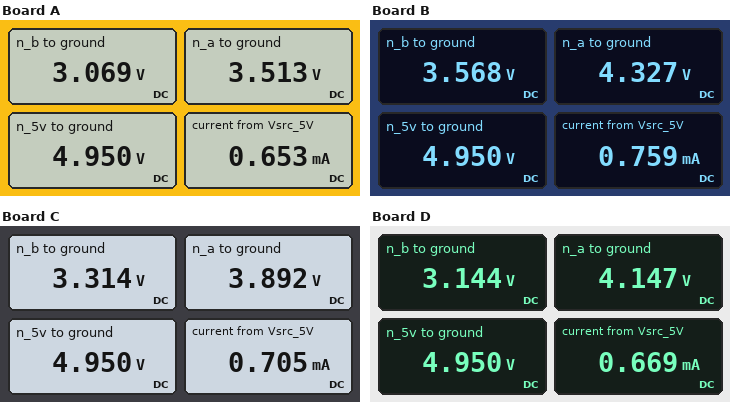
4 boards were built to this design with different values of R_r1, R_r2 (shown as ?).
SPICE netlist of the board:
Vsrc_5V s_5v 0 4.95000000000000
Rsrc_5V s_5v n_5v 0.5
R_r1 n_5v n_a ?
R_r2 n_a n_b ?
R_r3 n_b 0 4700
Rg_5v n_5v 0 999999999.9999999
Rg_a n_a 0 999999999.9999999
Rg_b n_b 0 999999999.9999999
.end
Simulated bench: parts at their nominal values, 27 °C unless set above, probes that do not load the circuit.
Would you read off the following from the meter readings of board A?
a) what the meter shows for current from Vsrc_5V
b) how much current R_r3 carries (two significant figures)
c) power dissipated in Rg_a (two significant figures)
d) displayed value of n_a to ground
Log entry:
0.653 mA
650 µA
12 nW
3.513 V
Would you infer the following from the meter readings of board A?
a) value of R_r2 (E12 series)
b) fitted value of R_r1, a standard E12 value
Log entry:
680 Ω
2.2 kΩ
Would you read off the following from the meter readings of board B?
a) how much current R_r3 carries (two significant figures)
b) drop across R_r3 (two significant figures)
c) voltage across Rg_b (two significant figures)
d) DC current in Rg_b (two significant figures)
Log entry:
760 µA
3.6 V
3.6 V
3.6 nA
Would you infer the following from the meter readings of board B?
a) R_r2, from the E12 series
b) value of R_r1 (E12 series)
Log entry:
1 kΩ
820 Ω
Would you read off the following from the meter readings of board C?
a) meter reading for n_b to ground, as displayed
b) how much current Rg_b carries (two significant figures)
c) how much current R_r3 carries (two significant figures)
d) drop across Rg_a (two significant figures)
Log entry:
3.314 V
3.3 nA
710 µA
3.9 V
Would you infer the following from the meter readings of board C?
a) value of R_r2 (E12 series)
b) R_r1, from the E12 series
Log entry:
820 Ω
1.5 kΩ
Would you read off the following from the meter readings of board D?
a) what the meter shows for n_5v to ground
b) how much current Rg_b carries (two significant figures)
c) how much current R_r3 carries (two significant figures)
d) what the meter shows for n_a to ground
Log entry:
4.950 V
3.1 nA
670 µA
4.147 V
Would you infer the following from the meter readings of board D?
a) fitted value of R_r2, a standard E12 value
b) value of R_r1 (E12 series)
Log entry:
1.5 kΩ
1.2 kΩ
